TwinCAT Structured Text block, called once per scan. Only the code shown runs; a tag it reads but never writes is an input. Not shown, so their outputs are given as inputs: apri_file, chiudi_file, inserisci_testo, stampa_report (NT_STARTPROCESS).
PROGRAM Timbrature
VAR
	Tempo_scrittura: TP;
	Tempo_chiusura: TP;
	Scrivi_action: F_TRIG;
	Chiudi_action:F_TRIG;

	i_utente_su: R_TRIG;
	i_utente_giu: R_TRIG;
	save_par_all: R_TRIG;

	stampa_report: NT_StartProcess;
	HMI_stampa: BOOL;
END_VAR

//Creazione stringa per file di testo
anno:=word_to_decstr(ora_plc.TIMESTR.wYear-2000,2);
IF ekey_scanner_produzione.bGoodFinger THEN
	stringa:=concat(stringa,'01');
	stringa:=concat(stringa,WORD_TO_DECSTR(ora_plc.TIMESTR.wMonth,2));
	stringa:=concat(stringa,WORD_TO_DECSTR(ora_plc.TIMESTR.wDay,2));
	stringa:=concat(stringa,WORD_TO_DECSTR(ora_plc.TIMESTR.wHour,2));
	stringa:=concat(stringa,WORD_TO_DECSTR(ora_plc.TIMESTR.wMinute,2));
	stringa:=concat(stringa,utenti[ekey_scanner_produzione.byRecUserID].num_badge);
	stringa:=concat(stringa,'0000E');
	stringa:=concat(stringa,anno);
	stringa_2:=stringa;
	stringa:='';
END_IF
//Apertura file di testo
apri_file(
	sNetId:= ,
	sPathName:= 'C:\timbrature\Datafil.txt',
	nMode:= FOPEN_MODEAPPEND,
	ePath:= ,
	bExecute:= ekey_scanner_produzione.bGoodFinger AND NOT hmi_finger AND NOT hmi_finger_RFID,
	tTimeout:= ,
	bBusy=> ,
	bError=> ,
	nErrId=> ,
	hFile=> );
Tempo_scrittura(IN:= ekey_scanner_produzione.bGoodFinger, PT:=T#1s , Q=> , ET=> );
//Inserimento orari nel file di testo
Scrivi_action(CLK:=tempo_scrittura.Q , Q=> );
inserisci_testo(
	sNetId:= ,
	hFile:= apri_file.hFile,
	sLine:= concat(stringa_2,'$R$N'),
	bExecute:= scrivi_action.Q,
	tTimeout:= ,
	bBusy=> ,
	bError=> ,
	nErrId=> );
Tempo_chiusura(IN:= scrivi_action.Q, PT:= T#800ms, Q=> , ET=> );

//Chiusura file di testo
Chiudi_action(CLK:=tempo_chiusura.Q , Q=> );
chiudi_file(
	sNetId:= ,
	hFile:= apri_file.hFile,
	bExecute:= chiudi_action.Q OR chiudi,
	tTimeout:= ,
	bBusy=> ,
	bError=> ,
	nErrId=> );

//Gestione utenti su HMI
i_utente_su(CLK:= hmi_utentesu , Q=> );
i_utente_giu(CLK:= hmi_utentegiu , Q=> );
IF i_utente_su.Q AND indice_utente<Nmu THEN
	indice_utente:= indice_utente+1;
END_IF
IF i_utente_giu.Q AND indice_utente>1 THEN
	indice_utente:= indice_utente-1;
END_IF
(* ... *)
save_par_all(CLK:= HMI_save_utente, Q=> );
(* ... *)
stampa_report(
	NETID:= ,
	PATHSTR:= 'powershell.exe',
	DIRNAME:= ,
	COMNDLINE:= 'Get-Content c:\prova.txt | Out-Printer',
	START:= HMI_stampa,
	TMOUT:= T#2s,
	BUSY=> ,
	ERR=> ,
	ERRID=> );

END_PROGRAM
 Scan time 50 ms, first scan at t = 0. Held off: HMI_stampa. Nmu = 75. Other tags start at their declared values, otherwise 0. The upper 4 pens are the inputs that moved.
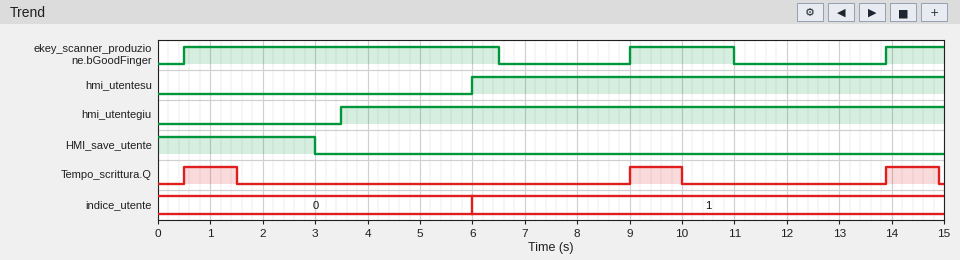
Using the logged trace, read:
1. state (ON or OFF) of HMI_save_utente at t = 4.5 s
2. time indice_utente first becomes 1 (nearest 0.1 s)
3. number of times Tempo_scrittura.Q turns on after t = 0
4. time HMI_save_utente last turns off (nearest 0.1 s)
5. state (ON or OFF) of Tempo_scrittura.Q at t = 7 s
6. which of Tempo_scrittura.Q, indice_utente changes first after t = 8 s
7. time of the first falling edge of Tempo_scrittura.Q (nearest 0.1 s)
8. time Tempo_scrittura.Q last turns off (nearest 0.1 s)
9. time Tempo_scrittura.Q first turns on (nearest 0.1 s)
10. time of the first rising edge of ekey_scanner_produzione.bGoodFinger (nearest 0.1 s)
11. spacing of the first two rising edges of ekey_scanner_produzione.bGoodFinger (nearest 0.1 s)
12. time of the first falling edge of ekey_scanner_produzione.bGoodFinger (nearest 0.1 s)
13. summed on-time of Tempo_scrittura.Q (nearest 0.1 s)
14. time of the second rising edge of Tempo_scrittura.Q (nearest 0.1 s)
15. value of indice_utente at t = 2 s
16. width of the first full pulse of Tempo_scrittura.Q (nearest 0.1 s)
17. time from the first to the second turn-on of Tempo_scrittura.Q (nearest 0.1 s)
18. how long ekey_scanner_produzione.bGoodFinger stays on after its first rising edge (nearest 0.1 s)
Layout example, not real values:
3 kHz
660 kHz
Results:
OFF
6.0 s
3
3.0 s
OFF
Tempo_scrittura.Q
1.5 s
14.9 s
0.5 s
0.5 s
8.5 s
6.5 s
3.0 s
9.0 s
0
1.0 s
8.5 s
6.0 s
